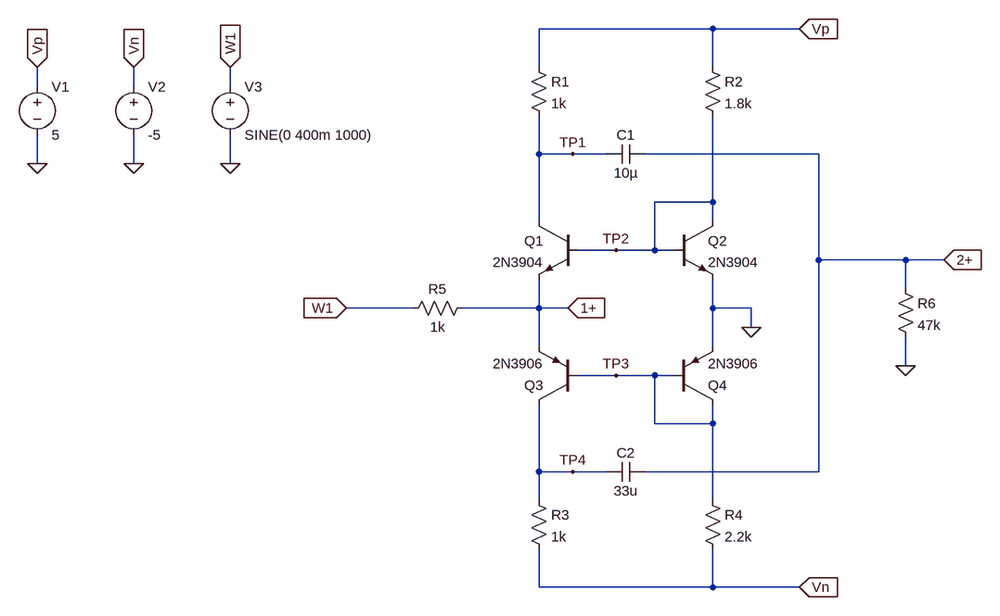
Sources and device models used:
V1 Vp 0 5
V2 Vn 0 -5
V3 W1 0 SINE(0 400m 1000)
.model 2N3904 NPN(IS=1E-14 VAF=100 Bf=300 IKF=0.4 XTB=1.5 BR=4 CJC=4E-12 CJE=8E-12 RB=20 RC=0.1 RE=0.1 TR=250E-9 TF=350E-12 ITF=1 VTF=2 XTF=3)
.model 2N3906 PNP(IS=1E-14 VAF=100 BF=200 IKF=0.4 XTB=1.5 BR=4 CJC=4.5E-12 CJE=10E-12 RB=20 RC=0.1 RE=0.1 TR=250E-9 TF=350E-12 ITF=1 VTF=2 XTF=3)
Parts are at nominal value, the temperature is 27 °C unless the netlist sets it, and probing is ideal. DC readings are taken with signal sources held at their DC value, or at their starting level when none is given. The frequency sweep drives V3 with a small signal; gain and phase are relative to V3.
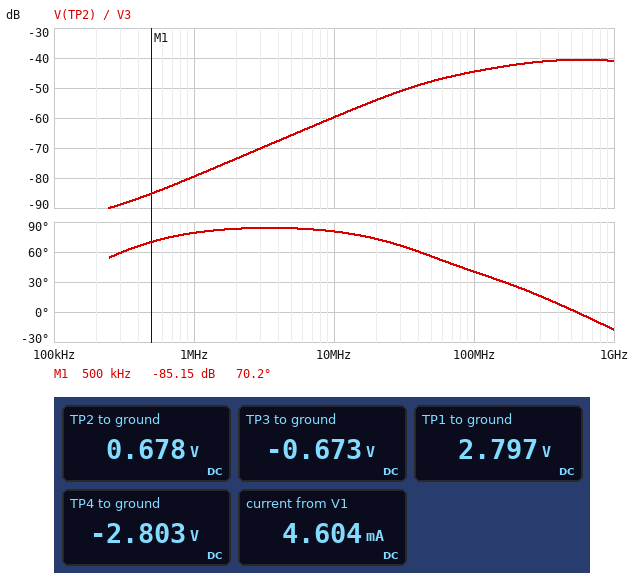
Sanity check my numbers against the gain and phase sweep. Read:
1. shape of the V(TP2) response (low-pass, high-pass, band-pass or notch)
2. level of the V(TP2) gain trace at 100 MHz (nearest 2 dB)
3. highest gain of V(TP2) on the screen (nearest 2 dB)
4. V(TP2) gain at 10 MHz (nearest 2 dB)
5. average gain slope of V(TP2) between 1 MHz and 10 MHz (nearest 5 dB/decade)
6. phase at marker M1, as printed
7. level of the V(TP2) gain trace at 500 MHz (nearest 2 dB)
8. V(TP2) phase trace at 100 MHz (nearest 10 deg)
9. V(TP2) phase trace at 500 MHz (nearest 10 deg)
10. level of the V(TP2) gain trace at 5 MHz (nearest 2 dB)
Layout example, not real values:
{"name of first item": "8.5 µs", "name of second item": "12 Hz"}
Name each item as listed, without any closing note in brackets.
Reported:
{"shape of the V(TP2) response": "high-pass", "level of the V(TP2) gain trace at 100 MHz": "-44 dB", "highest gain of V(TP2) on the screen": "-40 dB", "V(TP2) gain at 10 MHz": "-60 dB", "average gain slope of V(TP2) between 1 MHz and 10 MHz": "20 dB/decade", "phase at marker M1, as printed": "70.2 deg", "level of the V(TP2) gain trace at 500 MHz": "-40 dB", "V(TP2) phase trace at 100 MHz": "40 deg", "V(TP2) phase trace at 500 MHz": "0 deg", "level of the V(TP2) gain trace at 5 MHz": "-66 dB"}
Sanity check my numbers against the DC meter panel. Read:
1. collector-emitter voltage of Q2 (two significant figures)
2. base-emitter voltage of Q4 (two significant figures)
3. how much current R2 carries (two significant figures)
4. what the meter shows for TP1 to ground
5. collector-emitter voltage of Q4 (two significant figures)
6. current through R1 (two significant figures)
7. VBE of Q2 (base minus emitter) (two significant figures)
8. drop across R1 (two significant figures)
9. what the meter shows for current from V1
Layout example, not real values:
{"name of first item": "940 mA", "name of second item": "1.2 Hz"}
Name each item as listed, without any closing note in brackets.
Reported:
{"collector-emitter voltage of Q2": "680 mV", "base-emitter voltage of Q4": "-670 mV", "how much current R2 carries": "2.4 mA", "what the meter shows for TP1 to ground": "2.797 V", "collector-emitter voltage of Q4": "-670 mV", "current through R1": "2.2 mA", "VBE of Q2 (base minus emitter)": "680 mV", "drop across R1": "2.2 V", "what the meter shows for current from V1": "4.604 mA"}
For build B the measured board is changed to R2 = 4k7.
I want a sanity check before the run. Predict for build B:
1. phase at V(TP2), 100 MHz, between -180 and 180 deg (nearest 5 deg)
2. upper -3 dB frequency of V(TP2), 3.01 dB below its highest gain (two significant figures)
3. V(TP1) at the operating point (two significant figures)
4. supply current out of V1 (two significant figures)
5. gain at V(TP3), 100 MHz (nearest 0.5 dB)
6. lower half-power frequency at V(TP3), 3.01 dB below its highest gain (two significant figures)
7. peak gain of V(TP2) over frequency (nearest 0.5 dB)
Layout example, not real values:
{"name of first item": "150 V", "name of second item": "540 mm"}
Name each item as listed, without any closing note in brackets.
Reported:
{"phase at V(TP2), 100 MHz, between -180 and 180 deg": "20 deg", "upper -3 dB frequency of V(TP2), 3.01 dB below its highest gain": "1.7 GHz", "V(TP1) at the operating point": "3.6 V", "supply current out of V1": "2.3 mA", "gain at V(TP3), 100 MHz": "-42.0 dB", "lower half-power frequency at V(TP3), 3.01 dB below its highest gain": "80 MHz", "peak gain of V(TP2) over frequency": "-38.5 dB"}
